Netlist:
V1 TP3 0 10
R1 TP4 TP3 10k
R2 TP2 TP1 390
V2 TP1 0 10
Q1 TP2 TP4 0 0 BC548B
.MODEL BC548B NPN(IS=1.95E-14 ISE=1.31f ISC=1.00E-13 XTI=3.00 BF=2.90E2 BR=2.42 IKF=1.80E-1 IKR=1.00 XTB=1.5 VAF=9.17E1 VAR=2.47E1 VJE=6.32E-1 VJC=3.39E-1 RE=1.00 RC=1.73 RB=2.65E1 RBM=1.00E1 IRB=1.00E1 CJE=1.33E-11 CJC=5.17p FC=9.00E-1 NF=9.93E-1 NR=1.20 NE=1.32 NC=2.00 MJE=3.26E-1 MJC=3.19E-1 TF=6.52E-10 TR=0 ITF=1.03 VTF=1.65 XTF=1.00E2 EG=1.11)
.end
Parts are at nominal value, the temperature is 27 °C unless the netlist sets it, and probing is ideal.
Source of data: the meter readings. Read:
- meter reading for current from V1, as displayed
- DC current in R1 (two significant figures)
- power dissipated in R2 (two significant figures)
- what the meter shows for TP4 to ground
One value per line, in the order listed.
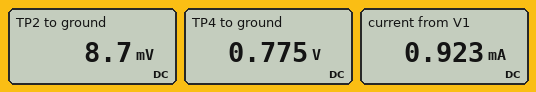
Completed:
0.923 mA
920 µA
260 mW
0.775 V
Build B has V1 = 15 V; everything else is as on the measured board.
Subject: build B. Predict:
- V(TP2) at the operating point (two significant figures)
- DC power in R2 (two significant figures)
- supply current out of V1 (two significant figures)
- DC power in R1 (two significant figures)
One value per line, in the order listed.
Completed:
-4.0 mV
260 mW
1.4 mA
20 mW
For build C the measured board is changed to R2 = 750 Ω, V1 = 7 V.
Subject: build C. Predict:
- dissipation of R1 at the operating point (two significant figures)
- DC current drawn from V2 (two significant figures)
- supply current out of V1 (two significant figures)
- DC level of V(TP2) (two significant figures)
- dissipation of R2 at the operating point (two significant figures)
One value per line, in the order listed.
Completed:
3.9 mW
13 mA
630 µA
-32 mV
130 mW
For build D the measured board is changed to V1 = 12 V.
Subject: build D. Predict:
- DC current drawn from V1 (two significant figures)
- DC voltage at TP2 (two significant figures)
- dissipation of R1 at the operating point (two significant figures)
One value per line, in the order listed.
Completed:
1.1 mA
2.8 mV
13 mW
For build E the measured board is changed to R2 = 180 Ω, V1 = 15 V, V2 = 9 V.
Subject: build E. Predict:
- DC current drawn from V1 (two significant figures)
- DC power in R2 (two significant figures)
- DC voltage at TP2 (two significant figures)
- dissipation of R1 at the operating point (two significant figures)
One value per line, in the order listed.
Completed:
1.4 mA
440 mW
82 mV
20 mW
